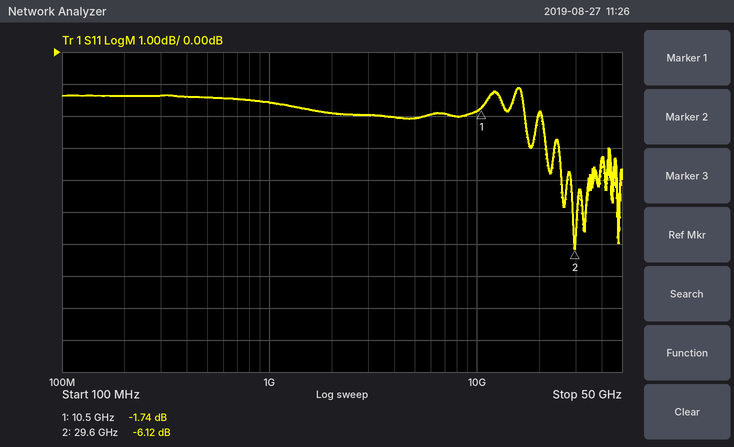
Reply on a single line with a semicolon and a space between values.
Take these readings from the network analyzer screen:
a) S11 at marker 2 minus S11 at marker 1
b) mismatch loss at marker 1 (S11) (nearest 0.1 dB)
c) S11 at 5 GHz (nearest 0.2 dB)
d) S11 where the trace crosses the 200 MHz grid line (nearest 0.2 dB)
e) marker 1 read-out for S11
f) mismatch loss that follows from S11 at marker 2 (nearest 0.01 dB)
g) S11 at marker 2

-4.38 dB; 4.8 dB; -2.0 dB; -1.4 dB; -1.74 dB; 1.22 dB; -6.12 dB
